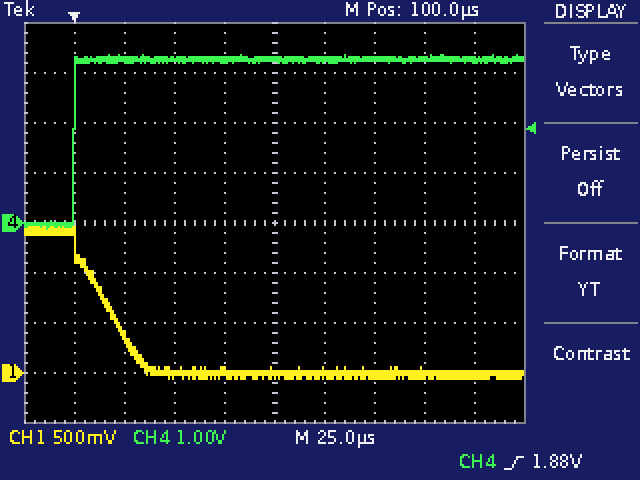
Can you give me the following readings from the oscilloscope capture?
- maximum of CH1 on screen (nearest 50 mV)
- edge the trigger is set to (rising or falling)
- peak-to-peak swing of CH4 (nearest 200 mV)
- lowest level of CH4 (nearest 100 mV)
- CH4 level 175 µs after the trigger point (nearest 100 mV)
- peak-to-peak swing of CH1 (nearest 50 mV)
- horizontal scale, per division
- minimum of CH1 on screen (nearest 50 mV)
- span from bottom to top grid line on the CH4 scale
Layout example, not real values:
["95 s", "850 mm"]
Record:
["1.45 V", "rising", "3.4 V", "-100 mV", "3.3 V", "1.50 V", "25 µs", "-50 mV", "8 V"]
